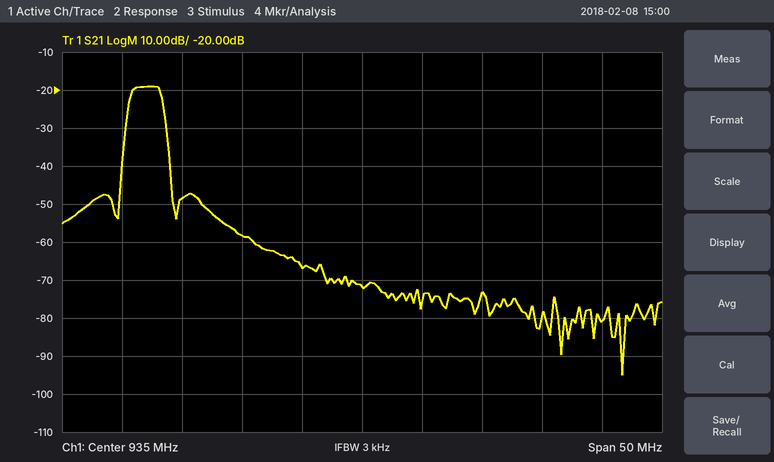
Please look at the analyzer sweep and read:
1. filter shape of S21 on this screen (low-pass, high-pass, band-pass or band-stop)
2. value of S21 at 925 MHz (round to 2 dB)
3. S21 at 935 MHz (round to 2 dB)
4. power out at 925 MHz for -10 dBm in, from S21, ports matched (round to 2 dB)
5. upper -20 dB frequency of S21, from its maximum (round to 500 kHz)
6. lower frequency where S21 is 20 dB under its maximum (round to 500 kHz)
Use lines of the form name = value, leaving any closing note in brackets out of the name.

filter shape of S21 on this screen = band-pass
value of S21 at 925 MHz = -58 dB
S21 at 935 MHz = -72 dB
power out at 925 MHz for -10 dBm in, from S21, ports matched = -68 dBm
upper -20 dB frequency of S21, from its maximum = 919.0 MHz
lower frequency where S21 is 20 dB under its maximum = 915.0 MHz
